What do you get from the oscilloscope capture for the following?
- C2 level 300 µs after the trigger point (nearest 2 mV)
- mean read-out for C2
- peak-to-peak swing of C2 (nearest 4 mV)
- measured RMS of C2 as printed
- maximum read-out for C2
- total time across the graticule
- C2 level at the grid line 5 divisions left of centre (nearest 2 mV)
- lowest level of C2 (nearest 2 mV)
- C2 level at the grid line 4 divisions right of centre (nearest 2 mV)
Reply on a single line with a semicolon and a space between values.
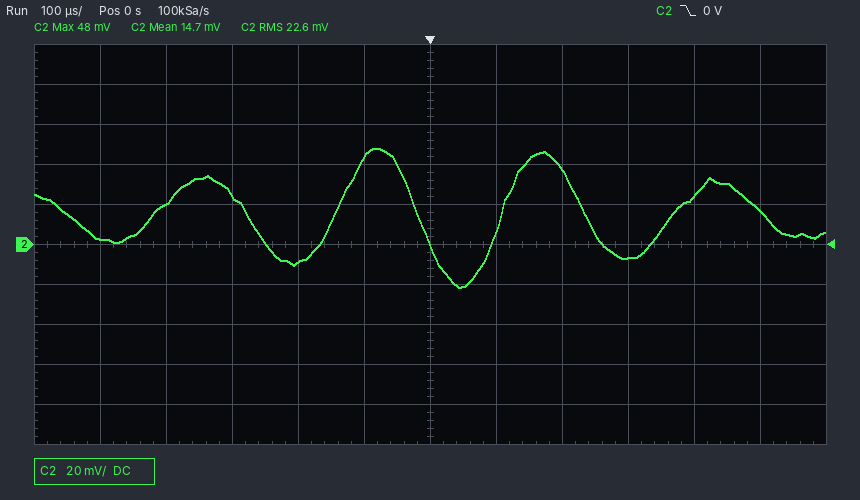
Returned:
-6 mV; 14.7 mV; 68 mV; 22.6 mV; 48 mV; 1.2 ms; 2 mV; -22 mV; 24 mV
